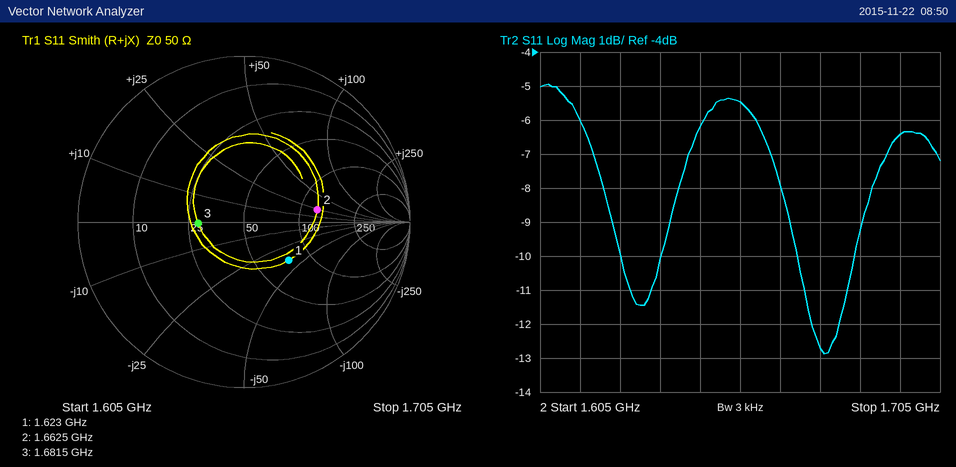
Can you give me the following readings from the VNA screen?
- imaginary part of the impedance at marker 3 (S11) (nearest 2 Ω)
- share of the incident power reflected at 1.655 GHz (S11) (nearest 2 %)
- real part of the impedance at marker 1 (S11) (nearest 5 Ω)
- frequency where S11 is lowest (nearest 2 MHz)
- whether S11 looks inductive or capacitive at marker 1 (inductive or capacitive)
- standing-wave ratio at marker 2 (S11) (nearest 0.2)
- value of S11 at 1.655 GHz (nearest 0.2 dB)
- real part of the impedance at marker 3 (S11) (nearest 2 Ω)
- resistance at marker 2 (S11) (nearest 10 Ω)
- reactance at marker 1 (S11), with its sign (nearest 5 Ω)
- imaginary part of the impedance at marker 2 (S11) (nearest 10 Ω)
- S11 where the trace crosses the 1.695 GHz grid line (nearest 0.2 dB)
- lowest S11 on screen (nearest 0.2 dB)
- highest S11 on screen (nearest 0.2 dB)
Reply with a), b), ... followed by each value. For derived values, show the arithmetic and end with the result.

a) 0 Ω
b) 10^(-5.4/10) ≈ 28.8 %, so 28 % to the nearest 2 %
c) 75 Ω
d) 1.676 GHz
e) capacitive
f) 2.6
g) -5.4 dB
h) 28 Ω
i) 130 Ω
j) -40 Ω
k) +20 Ω
l) -6.4 dB
m) -12.8 dB
n) -5.0 dB
